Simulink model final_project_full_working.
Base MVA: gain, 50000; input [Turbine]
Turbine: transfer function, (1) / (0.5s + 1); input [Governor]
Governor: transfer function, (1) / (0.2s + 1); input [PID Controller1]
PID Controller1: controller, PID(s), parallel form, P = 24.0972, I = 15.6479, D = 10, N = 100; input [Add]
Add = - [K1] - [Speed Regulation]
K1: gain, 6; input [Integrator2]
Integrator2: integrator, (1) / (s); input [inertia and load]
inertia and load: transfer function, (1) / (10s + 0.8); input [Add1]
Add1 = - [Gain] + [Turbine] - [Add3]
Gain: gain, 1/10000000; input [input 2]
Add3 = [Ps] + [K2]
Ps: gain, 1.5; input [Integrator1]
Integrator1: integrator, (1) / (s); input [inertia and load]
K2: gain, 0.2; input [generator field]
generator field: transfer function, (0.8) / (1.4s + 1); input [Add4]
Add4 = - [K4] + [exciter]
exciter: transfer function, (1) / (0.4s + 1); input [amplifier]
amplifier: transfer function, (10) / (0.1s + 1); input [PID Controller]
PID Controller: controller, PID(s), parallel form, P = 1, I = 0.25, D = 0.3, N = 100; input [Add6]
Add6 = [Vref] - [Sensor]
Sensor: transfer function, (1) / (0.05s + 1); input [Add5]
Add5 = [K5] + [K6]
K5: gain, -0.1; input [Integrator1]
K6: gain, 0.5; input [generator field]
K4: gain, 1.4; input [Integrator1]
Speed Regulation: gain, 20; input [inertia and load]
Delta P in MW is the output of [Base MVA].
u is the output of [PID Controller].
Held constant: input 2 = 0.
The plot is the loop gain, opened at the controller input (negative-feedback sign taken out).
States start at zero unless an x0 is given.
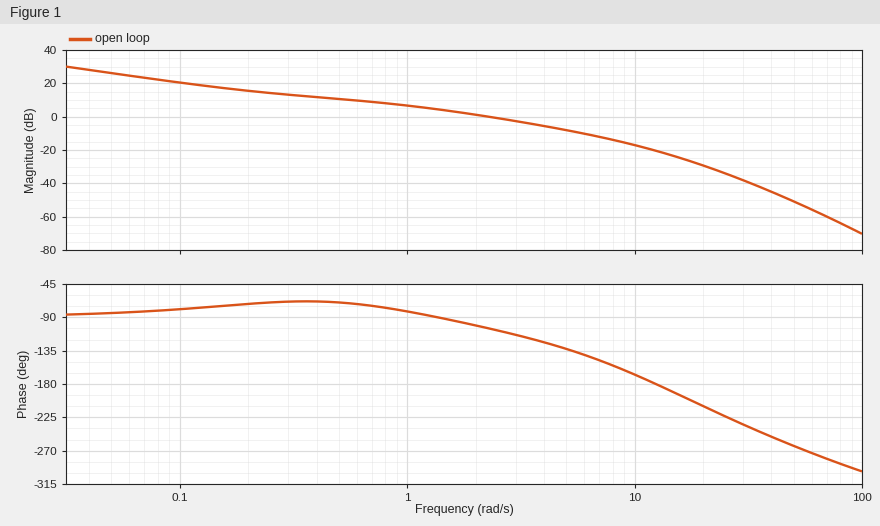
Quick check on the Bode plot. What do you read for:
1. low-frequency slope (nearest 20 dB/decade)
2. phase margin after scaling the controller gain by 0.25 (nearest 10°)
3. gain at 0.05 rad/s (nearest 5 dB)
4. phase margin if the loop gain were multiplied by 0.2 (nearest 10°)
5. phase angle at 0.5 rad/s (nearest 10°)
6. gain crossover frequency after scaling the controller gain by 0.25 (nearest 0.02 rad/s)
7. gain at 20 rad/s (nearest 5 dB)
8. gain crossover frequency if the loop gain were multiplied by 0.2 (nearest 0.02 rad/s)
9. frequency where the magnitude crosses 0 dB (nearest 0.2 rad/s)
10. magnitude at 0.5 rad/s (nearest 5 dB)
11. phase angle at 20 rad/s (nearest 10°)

-20 dB/decade
110°
25 dB
110°
-70°
0.38 rad/s
-30 dB
0.26 rad/s
2.2 rad/s
10 dB
-210°
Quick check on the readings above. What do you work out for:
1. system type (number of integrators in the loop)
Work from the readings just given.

1
